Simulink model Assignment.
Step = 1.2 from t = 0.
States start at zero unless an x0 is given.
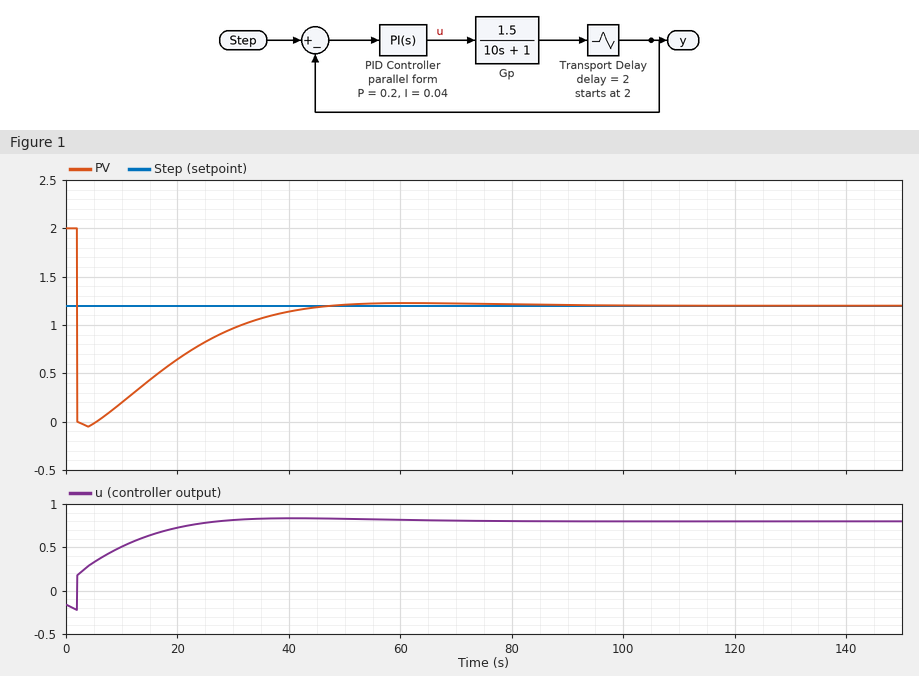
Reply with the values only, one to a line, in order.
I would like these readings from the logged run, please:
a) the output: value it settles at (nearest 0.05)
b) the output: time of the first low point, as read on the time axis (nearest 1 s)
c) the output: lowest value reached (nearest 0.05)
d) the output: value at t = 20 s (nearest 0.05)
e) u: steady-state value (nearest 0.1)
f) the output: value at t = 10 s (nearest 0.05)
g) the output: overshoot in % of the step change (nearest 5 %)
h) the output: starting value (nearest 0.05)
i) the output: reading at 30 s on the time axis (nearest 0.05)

1.20
4 s
-0.05
0.65
0.8
0.20
155 %
2.00
0.95
